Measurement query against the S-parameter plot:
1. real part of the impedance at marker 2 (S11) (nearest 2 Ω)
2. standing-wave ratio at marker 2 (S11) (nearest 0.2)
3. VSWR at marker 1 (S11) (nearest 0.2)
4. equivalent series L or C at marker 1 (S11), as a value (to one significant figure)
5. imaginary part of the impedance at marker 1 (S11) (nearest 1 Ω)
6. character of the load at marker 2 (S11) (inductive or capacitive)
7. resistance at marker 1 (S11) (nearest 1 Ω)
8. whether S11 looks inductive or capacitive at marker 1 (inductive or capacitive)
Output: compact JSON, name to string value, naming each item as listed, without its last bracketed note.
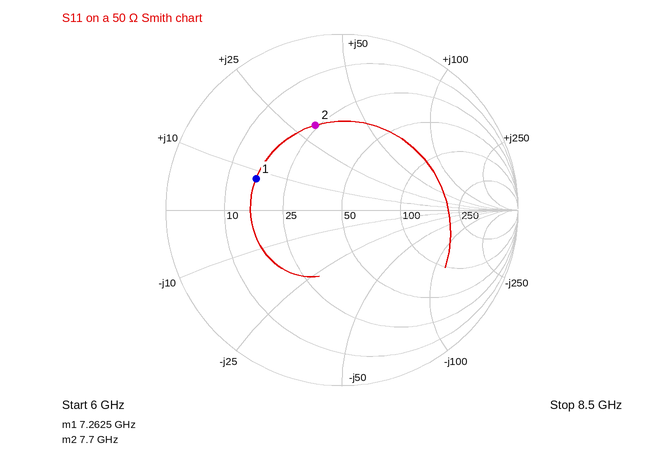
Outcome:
{"real part of the impedance at marker 2 (S11)": "24 Ω", "standing-wave ratio at marker 2 (S11)": "3.0", "VSWR at marker 1 (S11)": "3.2", "equivalent series L or C at marker 1 (S11), as a value": "200 pH", "imaginary part of the impedance at marker 1 (S11)": "+8 Ω", "character of the load at marker 2 (S11)": "inductive", "resistance at marker 1 (S11)": "16 Ω", "whether S11 looks inductive or capacitive at marker 1": "inductive"}
